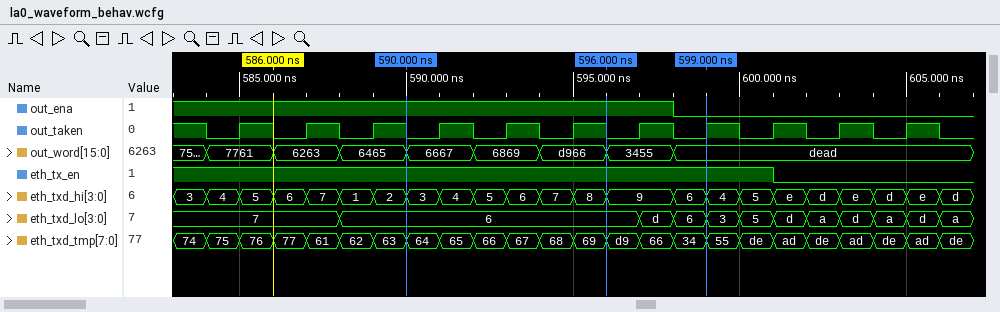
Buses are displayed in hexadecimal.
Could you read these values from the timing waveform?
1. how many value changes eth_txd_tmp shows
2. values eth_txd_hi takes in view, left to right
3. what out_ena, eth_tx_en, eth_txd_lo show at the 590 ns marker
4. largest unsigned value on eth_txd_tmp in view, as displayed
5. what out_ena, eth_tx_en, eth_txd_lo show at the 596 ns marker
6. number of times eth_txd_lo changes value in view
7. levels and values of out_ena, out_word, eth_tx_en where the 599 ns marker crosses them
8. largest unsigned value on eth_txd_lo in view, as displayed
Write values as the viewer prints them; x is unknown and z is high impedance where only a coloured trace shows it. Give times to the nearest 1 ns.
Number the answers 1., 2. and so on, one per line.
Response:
1. 23
2. 3, 4, 5, 6, 7, 1, 2, 3, 4, 5, 6, 7, 8, 9, 6, 4, 5, e, d, e, d, e, d
3. out_ena=1, eth_tx_en=1, eth_txd_lo=6
4. de
5. out_ena=1, eth_tx_en=1, eth_txd_lo=6
6. 11
7. out_ena=0, out_word=dead, eth_tx_en=1
8. d
